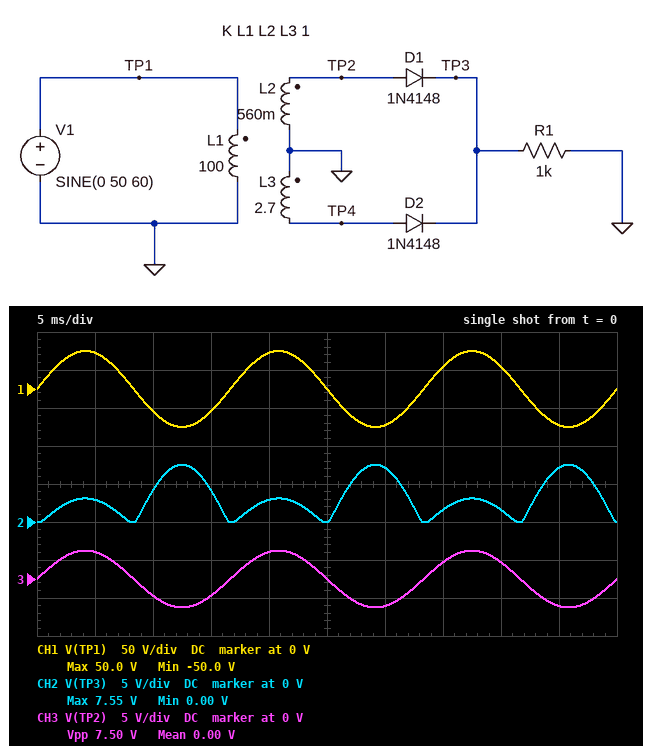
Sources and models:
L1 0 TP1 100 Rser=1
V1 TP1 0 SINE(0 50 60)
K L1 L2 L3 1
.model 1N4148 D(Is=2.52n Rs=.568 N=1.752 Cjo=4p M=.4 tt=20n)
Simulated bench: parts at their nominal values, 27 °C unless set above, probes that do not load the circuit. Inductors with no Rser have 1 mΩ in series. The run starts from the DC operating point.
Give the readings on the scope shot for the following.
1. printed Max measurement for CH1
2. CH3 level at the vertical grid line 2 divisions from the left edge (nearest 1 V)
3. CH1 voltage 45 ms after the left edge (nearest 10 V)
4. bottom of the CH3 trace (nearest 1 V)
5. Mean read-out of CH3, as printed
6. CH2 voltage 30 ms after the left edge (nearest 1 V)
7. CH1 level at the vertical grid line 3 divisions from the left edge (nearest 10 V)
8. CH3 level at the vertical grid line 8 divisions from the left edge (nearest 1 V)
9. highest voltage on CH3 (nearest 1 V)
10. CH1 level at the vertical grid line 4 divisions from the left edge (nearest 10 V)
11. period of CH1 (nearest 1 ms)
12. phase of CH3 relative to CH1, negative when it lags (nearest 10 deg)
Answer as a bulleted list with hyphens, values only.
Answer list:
- 50.0 V
- -2 V
- -50 V
- -4 V
- 0.00 V
- 7 V
- -30 V
- 2 V
- 4 V
- 50 V
- 17 ms
- 0 deg
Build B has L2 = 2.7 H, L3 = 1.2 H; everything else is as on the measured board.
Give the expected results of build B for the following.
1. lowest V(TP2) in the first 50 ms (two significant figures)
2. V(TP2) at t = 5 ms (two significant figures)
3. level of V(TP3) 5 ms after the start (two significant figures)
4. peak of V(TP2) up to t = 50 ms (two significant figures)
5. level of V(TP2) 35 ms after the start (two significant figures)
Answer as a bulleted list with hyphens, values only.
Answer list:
- -8.2 V
- 7.8 V
- 7.1 V
- 8.2 V
- 4.8 V
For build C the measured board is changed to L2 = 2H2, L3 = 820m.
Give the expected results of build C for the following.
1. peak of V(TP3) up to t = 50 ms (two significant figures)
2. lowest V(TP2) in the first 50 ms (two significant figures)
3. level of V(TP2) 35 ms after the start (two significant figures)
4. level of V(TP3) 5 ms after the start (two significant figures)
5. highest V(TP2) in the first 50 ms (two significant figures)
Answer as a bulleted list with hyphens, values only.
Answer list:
- 6.7 V
- -7.4 V
- 4.4 V
- 6.4 V
- 7.4 V
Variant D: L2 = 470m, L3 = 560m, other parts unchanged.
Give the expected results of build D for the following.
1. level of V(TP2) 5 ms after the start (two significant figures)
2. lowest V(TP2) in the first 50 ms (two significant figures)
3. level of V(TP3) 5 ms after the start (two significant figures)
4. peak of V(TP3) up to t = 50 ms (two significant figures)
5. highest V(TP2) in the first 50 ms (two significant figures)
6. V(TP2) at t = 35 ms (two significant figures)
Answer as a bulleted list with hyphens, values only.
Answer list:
- 3.3 V
- -3.4 V
- 2.6 V
- 3.1 V
- 3.4 V
- 2.0 V
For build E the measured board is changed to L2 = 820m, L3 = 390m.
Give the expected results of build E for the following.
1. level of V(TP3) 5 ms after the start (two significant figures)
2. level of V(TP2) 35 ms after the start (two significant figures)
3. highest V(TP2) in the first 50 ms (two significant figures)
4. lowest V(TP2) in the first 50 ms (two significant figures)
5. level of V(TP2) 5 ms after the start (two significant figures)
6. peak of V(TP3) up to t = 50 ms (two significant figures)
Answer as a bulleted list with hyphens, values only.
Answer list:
- 3.7 V
- 2.7 V
- 4.5 V
- -4.5 V
- 4.3 V
- 3.9 V
